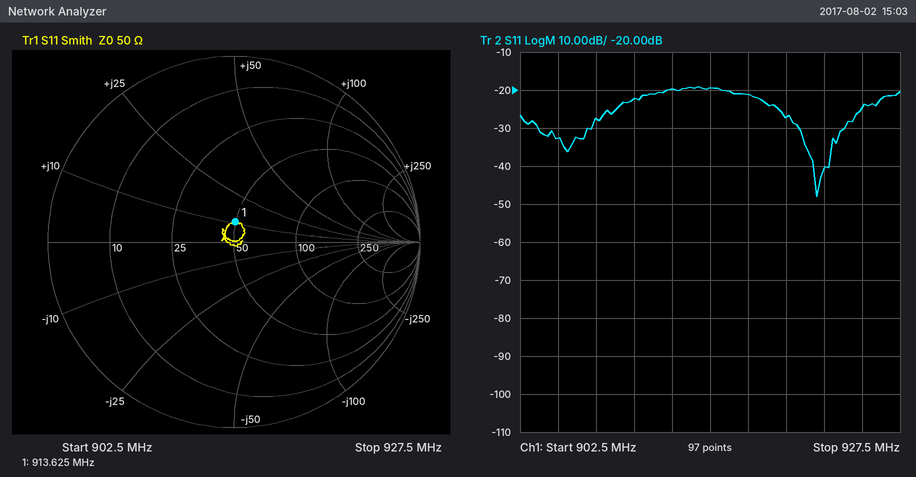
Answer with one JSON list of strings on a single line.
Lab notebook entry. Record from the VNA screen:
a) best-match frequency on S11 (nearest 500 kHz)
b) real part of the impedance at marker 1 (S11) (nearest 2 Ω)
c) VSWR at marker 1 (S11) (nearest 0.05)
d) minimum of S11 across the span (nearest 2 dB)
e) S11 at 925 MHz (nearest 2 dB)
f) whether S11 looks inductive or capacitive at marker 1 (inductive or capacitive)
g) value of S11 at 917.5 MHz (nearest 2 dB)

["922.0 MHz", "50 Ω", "1.25", "-48 dB", "-24 dB", "inductive", "-22 dB"]
